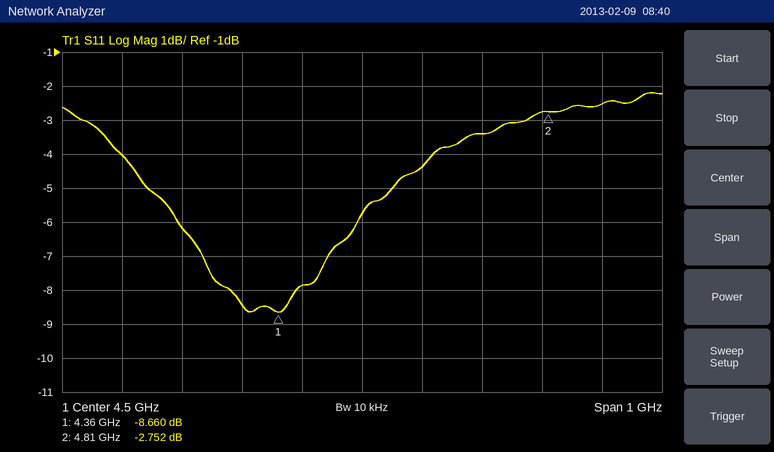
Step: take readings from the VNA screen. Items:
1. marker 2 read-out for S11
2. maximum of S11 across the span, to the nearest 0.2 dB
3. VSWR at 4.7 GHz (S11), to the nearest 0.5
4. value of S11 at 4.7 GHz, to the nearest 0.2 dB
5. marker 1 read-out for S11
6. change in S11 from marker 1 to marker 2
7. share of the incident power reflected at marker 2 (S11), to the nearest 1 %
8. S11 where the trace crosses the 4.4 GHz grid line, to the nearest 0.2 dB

-2.752 dB
-2.2 dB
5.0
-3.4 dB
-8.660 dB
5.908 dB
53 %
-7.8 dB
